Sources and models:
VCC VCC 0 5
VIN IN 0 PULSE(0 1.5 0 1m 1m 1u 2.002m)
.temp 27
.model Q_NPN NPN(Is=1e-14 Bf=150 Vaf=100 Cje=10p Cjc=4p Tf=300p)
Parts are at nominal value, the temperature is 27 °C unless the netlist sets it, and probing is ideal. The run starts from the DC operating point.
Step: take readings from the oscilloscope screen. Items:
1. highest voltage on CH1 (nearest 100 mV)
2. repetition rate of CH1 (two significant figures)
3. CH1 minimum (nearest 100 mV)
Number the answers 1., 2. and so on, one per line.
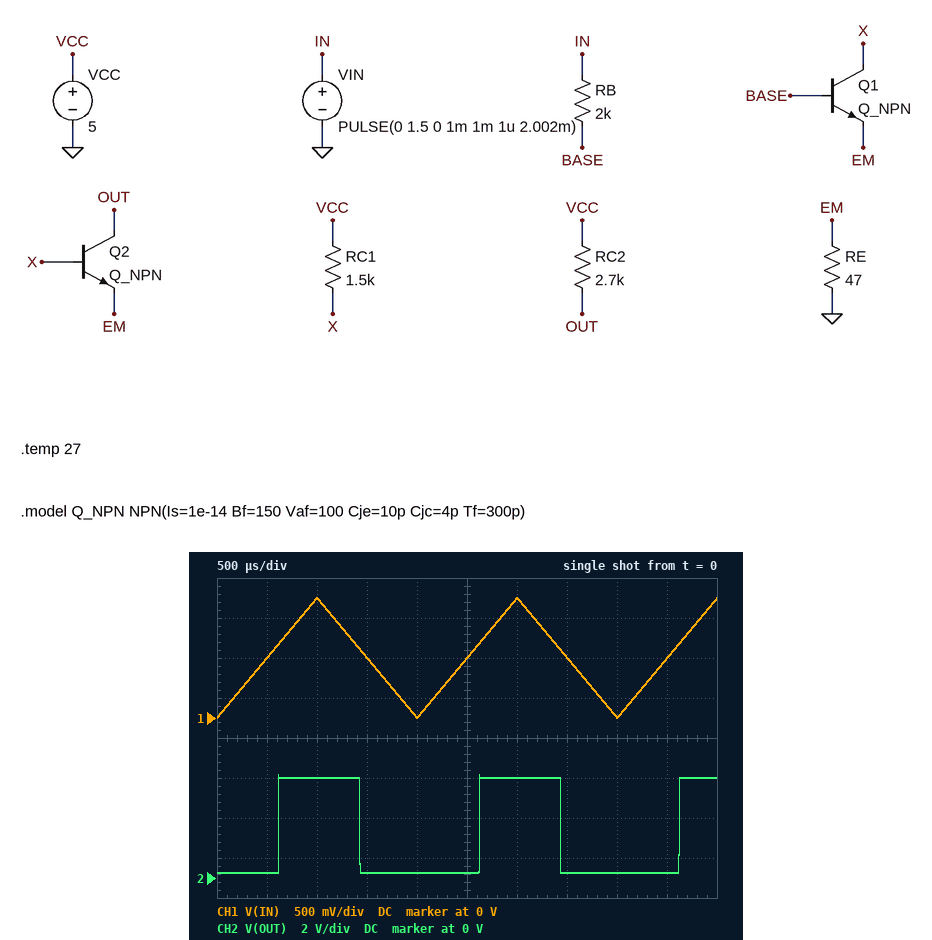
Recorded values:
1. 1.5 V
2. 500 Hz
3. 0 V
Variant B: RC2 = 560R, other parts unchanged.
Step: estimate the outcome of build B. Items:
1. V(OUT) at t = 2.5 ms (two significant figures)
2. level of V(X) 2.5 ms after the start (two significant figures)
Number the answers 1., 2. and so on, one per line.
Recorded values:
1. 540 mV
2. 1.2 V
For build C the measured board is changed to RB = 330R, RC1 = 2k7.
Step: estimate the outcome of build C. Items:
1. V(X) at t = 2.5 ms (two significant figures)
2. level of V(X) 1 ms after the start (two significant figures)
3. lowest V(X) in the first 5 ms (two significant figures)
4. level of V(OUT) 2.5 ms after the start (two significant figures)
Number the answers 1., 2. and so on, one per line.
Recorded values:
1. 850 mV
2. 200 mV
3. 150 mV
4. 190 mV
